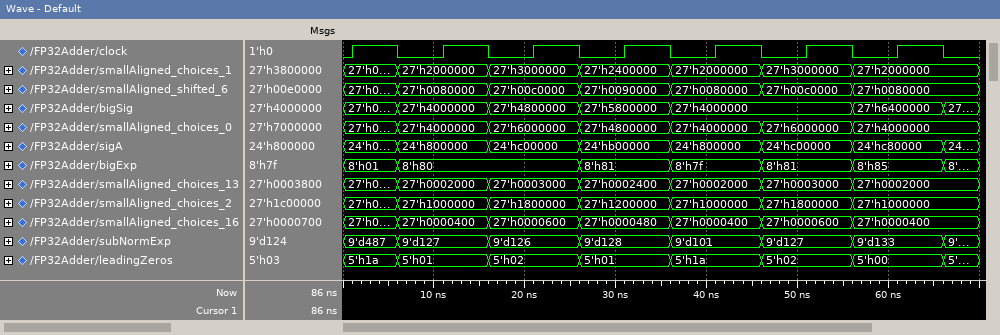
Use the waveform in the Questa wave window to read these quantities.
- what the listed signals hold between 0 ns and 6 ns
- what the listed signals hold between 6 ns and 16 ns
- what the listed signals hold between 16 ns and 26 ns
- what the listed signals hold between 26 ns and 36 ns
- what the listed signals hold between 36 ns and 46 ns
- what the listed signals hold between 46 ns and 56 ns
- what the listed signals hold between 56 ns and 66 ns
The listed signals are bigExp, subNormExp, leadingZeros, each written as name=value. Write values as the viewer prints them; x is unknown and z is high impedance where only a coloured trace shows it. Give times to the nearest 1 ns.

bigExp=8'h01, subNormExp=9'd487, leadingZeros=5'h1a
bigExp=8'h80, subNormExp=9'd127, leadingZeros=5'h01
bigExp=8'h80, subNormExp=9'd126, leadingZeros=5'h02
bigExp=8'h81, subNormExp=9'd128, leadingZeros=5'h01
bigExp=8'h7f, subNormExp=9'd101, leadingZeros=5'h1a
bigExp=8'h81, subNormExp=9'd127, leadingZeros=5'h02
bigExp=8'h85, subNormExp=9'd133, leadingZeros=5'h00
